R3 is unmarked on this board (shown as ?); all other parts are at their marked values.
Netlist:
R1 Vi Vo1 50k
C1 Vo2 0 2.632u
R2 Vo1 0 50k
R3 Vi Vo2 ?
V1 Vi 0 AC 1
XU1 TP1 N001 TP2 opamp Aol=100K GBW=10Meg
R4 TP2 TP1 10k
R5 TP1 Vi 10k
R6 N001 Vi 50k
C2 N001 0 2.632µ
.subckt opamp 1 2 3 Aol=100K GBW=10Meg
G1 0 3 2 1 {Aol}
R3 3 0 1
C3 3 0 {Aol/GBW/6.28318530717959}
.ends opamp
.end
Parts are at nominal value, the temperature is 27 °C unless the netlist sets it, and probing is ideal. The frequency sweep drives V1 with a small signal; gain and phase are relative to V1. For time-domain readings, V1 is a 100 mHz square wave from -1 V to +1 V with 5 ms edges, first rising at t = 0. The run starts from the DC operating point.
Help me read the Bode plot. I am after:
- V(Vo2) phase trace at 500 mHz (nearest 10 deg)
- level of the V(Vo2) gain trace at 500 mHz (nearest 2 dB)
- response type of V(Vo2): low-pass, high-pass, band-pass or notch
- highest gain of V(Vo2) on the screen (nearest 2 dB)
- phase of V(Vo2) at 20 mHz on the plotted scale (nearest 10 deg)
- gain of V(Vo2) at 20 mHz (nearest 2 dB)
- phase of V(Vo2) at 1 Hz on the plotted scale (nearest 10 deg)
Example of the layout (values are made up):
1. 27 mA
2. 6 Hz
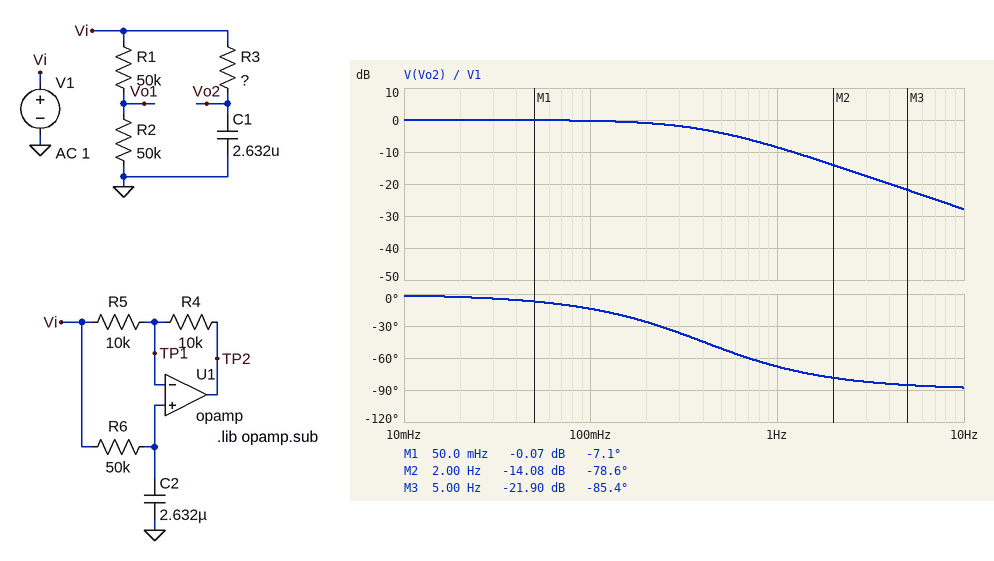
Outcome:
1. -50 deg
2. -4 dB
3. low-pass
4. 0 dB
5. 0 deg
6. 0 dB
7. -70 deg
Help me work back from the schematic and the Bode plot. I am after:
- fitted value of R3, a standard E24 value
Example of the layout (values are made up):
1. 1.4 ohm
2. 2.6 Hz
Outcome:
1. 150 kΩ
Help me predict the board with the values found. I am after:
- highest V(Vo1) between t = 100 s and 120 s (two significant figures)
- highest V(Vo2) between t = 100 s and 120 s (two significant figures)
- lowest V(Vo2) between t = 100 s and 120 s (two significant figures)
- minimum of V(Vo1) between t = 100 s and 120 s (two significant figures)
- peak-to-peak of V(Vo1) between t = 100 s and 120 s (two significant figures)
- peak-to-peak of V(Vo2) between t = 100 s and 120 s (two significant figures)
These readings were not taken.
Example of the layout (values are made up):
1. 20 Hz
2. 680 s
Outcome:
1. 500 mV
2. 1.0 V
3. -1.0 V
4. -500 mV
5. 1.0 V
6. 2.0 V
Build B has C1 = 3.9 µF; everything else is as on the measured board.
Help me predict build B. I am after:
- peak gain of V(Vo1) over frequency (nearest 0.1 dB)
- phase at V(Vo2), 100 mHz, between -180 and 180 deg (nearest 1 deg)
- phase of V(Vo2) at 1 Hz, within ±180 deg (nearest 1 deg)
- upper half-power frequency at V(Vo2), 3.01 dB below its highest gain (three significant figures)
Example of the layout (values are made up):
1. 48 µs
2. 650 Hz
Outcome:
1. -6.0 dB
2. -20 deg
3. -75 deg
4. 272 mHz
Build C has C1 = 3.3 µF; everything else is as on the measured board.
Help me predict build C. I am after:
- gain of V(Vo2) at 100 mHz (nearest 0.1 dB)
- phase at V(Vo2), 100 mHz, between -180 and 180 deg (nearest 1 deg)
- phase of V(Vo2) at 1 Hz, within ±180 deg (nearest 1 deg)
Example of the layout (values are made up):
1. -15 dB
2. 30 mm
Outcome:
1. -0.4 dB
2. -17 deg
3. -72 deg
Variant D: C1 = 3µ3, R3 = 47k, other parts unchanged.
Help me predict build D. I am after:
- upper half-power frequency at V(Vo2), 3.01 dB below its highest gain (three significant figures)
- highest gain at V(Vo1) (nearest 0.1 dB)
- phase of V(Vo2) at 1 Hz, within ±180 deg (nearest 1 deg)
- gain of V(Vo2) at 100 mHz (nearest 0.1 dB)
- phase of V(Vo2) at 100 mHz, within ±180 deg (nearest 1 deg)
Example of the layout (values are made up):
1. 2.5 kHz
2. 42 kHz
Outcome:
1. 1.03 Hz
2. -6.0 dB
3. -44 deg
4. 0 dB
5. -6 deg
